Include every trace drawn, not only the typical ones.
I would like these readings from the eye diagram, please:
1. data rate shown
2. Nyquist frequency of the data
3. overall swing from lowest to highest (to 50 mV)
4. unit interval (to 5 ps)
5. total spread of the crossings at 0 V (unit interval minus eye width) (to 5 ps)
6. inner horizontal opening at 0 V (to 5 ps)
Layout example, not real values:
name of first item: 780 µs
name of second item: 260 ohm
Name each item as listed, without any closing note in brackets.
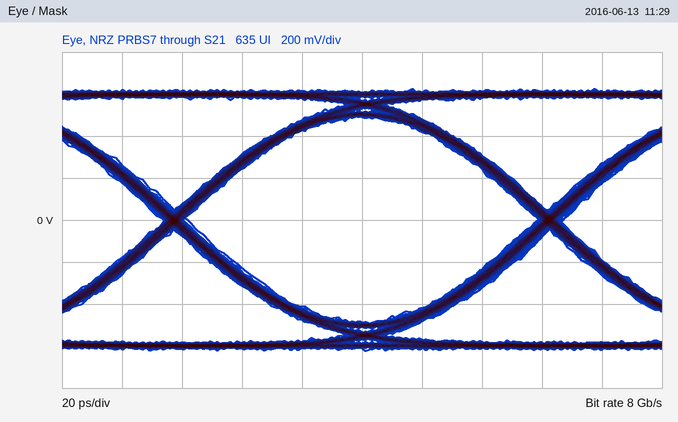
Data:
data rate shown: 8 Gb/s
Nyquist frequency of the data: 4 GHz
overall swing from lowest to highest: 1.25 V
unit interval: 125 ps
total spread of the crossings at 0 V (unit interval minus eye width): 10 ps
inner horizontal opening at 0 V: 115 ps
